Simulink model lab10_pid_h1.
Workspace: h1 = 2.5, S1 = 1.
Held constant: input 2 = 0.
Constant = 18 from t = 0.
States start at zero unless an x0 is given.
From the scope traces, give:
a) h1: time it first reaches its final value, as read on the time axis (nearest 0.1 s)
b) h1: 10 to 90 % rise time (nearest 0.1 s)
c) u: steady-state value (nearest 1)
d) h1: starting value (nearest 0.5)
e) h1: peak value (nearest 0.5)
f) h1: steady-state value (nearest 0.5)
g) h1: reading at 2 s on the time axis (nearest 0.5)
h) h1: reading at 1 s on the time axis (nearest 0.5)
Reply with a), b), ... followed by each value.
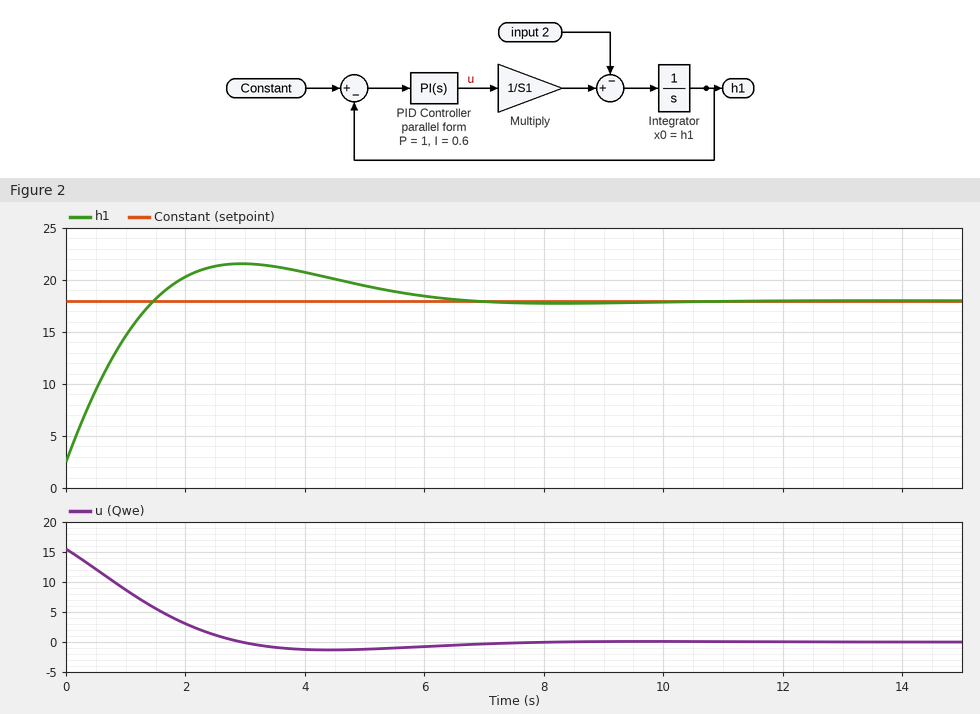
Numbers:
a) 1.5 s
b) 1.1 s
c) 0
d) 2.5
e) 21.5
f) 18.0
g) 20.5
h) 14.5
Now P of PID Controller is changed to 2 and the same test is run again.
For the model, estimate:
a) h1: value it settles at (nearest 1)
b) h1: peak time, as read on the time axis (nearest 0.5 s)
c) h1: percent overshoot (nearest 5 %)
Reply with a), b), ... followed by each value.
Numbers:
a) 18
b) 2.5 s
c) 10 %
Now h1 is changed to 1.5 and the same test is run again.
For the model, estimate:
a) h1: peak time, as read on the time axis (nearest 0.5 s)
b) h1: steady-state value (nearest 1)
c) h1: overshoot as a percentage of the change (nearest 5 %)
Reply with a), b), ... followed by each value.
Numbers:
a) 3.0 s
b) 18
c) 25 %
